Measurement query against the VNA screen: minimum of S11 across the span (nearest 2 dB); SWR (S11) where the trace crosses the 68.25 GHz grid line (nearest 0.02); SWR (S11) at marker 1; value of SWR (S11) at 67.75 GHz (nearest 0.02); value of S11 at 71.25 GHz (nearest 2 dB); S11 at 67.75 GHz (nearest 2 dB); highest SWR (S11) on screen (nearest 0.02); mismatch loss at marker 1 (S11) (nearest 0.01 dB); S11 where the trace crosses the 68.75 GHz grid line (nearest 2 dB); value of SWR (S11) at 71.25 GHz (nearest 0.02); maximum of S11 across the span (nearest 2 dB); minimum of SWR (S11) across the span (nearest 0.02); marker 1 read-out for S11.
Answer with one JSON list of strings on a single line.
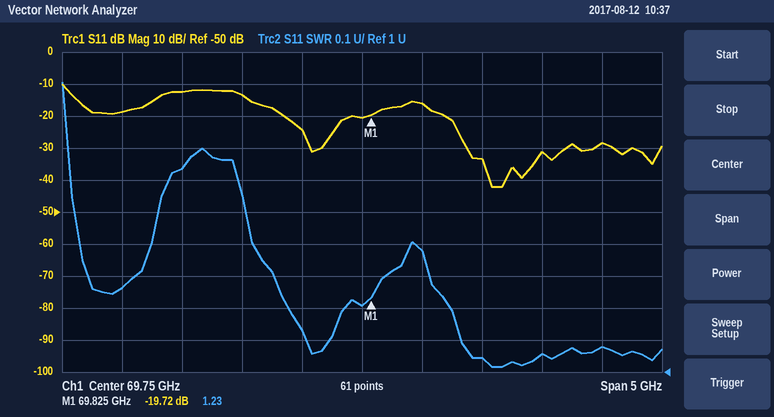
["-42 dB", "1.64", "1.23", "1.26", "-32 dB", "-18 dB", "1.90", "0.05 dB", "-14 dB", "1.06", "-10 dB", "1.02", "-19.72 dB"]
